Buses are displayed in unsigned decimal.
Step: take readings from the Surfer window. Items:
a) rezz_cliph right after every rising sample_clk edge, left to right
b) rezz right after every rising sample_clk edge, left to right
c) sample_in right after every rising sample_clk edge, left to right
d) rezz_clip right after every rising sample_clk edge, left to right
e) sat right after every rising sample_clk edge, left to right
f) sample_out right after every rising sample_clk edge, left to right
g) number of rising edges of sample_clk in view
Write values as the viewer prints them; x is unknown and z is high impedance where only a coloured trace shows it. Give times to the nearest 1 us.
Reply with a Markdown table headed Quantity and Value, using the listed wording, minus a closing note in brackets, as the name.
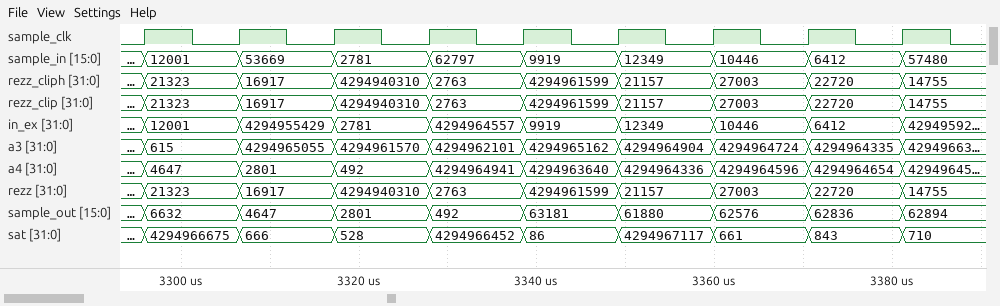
| Quantity | Value |
|---|---|
| rezz_cliph right after every rising sample_clk edge, left to right | 21323, 16917, 4294940310, 2763, 4294961599, 21157, 27003, 22720, 14755 |
| rezz right after every rising sample_clk edge, left to right | 21323, 16917, 4294940310, 2763, 4294961599, 21157, 27003, 22720, 14755 |
| sample_in right after every rising sample_clk edge, left to right | 12001, 53669, 2781, 62797, 9919, 12349, 10446, 6412, 57480 |
| rezz_clip right after every rising sample_clk edge, left to right | 21323, 16917, 4294940310, 2763, 4294961599, 21157, 27003, 22720, 14755 |
| sat right after every rising sample_clk edge, left to right | 4294966675, 666, 528, 4294966452, 86, 4294967117, 661, 843, 710 |
| sample_out right after every rising sample_clk edge, left to right | 6632, 4647, 2801, 492, 63181, 61880, 62576, 62836, 62894 |
| number of rising edges of sample_clk in view | 9 |
